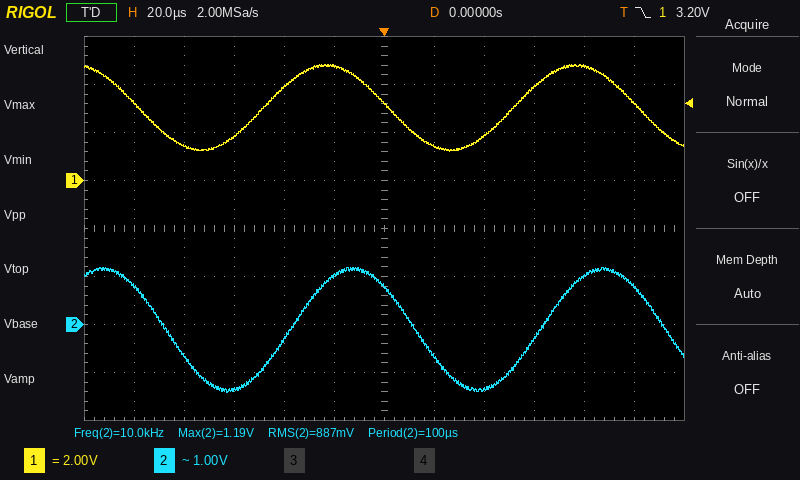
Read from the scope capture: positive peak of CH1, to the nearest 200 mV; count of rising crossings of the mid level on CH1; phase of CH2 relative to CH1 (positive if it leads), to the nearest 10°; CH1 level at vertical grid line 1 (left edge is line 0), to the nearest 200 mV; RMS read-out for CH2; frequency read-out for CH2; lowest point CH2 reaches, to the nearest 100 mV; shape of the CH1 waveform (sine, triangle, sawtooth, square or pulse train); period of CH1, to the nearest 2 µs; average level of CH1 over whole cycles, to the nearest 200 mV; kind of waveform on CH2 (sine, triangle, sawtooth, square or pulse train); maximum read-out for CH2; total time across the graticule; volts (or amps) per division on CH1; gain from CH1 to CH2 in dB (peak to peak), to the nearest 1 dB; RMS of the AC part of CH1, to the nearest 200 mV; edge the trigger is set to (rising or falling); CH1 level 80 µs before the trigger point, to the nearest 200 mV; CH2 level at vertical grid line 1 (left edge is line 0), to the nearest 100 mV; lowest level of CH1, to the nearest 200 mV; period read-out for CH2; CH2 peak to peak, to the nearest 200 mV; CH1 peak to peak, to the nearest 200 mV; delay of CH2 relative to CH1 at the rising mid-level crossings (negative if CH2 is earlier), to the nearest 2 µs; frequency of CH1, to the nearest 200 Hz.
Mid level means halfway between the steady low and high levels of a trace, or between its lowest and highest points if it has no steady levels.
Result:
4.8 V
2
-40°
3.2 V
887 mV
10.0 kHz
-1.4 V
sine
100 µs
3.0 V
sine
1.19 V
240 µs
2 V
-3 dB
1.2 V
falling
1.4 V
800 mV
1.2 V
100 µs
2.6 V
3.6 V
+10 µs
10.0 kHz
